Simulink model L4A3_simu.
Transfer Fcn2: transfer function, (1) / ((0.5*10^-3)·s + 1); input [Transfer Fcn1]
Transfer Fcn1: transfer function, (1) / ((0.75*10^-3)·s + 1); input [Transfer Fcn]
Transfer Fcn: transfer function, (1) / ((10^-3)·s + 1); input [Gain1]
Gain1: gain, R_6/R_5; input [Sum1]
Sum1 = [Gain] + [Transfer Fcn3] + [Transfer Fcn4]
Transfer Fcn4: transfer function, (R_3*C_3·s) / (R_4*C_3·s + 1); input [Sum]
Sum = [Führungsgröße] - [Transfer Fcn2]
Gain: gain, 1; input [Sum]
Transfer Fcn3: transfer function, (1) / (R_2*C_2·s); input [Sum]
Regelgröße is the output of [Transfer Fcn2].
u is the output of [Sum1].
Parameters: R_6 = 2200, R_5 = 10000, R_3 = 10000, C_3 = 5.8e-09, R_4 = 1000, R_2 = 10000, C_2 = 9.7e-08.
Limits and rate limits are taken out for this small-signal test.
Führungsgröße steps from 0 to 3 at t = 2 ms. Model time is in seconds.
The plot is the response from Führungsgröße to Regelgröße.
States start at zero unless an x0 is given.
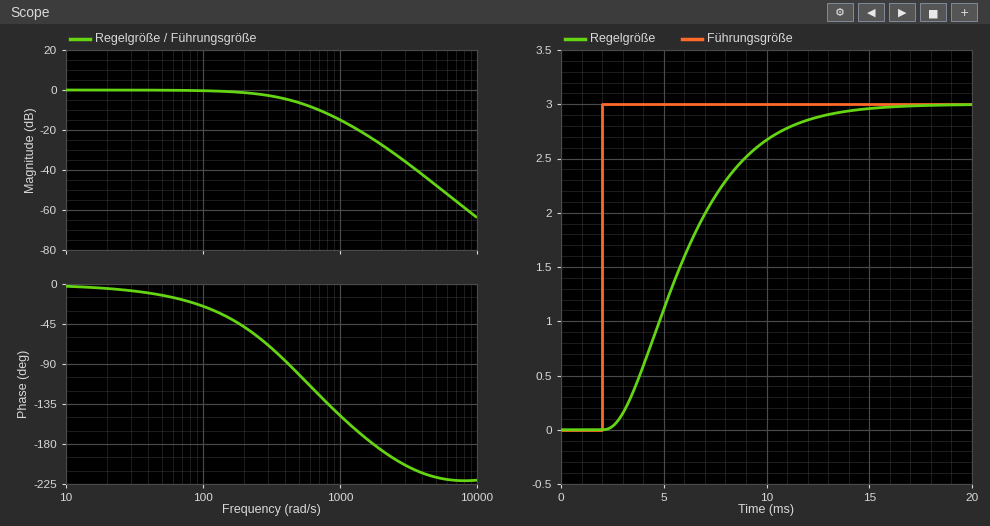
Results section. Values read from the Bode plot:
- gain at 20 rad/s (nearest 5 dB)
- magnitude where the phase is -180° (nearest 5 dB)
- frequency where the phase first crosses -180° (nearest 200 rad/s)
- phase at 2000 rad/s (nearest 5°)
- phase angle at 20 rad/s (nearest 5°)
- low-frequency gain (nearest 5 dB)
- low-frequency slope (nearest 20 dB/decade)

0 dB
-25 dB
1800 rad/s
-185°
-5°
0 dB
0 dB/decade
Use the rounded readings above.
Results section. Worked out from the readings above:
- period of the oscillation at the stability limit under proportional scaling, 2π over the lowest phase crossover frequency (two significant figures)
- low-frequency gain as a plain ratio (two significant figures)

0.0035 s
1.0
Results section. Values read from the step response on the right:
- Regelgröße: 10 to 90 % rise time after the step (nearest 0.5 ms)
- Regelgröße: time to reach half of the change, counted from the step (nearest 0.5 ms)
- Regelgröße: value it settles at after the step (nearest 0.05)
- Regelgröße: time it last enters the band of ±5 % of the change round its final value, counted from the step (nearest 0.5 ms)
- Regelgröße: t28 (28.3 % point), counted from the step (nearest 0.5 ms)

7.0 ms
4.0 ms
3.00
10.0 ms
2.5 ms
